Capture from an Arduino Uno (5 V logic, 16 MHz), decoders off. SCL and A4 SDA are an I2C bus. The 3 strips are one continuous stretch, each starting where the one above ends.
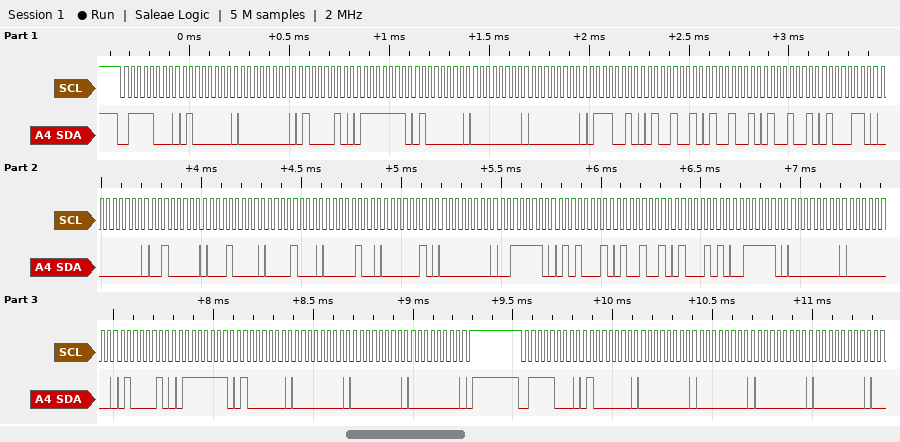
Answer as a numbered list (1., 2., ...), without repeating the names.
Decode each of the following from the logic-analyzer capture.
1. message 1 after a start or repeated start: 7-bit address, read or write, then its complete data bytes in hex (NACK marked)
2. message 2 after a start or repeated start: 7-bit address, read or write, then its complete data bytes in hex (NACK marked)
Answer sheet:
1. 0x3C write: 40 00 42 7F 40 00 00 72 49 49 49 46 00 20 10 08 04 02 00 3E 51 49 45 3E 00 00 42 7F 40 00 00 00
2. 0x3C write: 40 00 00 00 00
